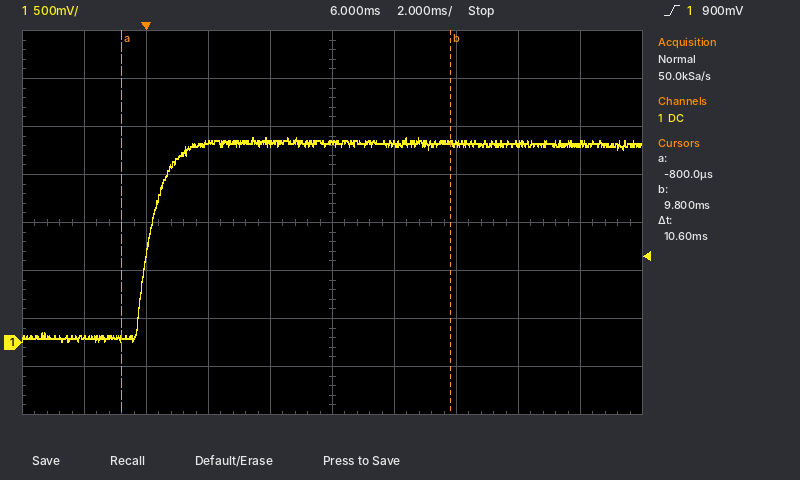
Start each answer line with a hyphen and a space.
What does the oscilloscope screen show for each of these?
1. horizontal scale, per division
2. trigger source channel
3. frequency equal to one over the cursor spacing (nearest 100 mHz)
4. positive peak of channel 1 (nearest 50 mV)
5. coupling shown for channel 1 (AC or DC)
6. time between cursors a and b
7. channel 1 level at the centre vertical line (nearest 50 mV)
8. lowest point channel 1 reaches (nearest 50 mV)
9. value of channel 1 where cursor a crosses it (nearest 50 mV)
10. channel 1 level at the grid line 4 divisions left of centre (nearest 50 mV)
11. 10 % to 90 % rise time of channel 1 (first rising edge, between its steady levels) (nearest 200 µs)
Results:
- 2 ms
- channel 1
- 94.3 Hz
- 2.15 V
- DC
- 10.6 ms
- 2.10 V
- 0 mV
- 50 mV
- 50 mV
- 1.2 ms
